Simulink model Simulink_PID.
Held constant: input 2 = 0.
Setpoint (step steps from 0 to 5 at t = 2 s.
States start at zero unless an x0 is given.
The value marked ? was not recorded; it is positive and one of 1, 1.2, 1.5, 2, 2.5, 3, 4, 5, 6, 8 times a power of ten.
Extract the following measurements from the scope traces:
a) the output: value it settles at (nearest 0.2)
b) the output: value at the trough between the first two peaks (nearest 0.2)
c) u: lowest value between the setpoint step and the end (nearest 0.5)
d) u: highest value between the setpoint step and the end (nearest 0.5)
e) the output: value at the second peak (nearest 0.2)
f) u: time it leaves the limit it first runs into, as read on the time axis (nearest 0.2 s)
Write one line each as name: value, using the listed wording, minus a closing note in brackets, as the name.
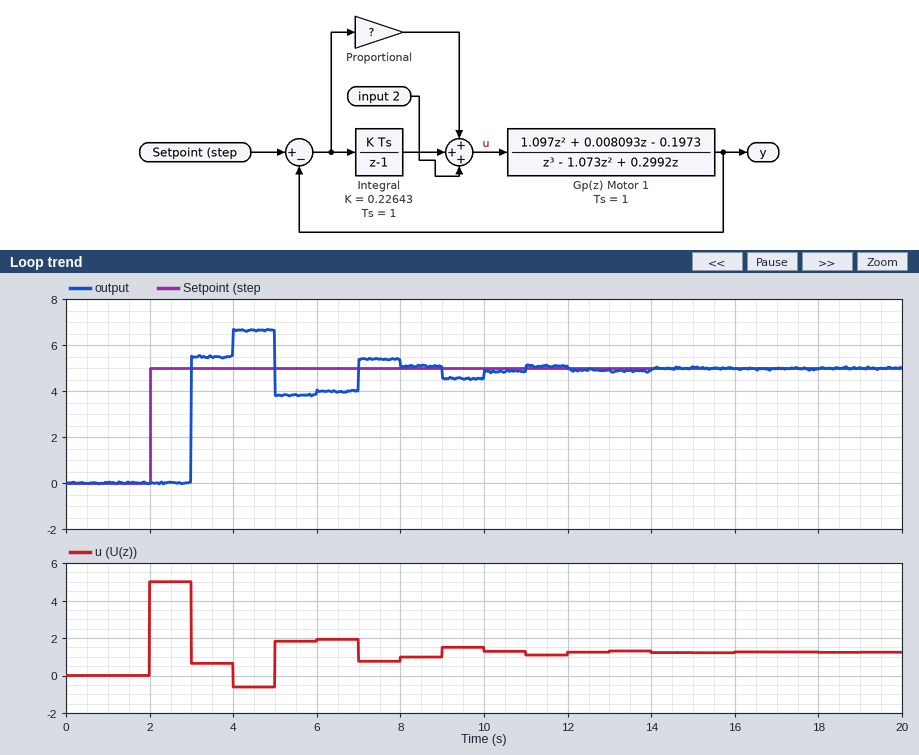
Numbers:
the output: value it settles at: 5.0
the output: value at the trough between the first two peaks: 3.8
u: lowest value between the setpoint step and the end: -0.5
u: highest value between the setpoint step and the end: 5.0
the output: value at the second peak: 5.4
u: time it leaves the limit it first runs into, as read on the time axis: 3.0 s
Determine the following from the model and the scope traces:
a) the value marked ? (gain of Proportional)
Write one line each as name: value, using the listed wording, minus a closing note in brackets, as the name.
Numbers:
the value marked ?: 1
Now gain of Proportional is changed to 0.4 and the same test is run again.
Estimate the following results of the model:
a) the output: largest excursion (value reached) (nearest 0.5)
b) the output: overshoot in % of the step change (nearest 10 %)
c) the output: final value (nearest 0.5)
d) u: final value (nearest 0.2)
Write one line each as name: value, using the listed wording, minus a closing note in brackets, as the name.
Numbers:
the output: largest excursion (value reached): 6.0
the output: overshoot in % of the step change: 20 %
the output: final value: 5.0
u: final value: 1.2
